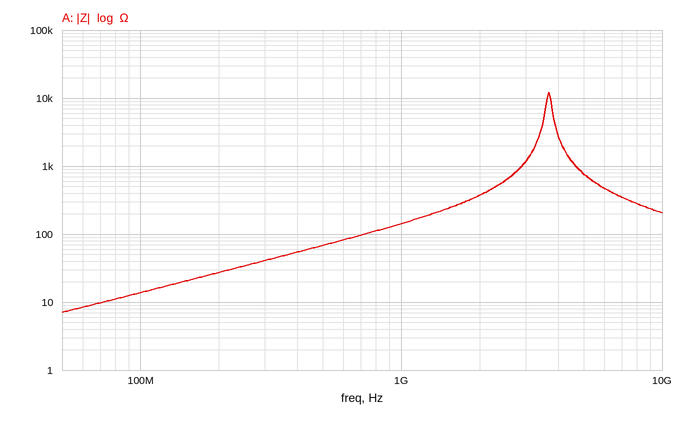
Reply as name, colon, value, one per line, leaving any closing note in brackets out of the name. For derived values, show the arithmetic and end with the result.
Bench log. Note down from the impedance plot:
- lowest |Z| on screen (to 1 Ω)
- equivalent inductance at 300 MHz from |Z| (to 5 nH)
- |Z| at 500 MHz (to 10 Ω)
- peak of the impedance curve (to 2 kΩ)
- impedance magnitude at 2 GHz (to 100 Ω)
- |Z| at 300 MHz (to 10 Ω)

lowest |Z| on screen: 7 Ω
equivalent inductance at 300 MHz from |Z|: L = 40 Ω/(2π × 300 MHz) ≈ 21.2 nH, so 20 nH to the nearest 5 nH
|Z| at 500 MHz: 70 Ω
peak of the impedance curve: 12 kΩ
impedance magnitude at 2 GHz: 400 Ω
|Z| at 300 MHz: 40 Ω
